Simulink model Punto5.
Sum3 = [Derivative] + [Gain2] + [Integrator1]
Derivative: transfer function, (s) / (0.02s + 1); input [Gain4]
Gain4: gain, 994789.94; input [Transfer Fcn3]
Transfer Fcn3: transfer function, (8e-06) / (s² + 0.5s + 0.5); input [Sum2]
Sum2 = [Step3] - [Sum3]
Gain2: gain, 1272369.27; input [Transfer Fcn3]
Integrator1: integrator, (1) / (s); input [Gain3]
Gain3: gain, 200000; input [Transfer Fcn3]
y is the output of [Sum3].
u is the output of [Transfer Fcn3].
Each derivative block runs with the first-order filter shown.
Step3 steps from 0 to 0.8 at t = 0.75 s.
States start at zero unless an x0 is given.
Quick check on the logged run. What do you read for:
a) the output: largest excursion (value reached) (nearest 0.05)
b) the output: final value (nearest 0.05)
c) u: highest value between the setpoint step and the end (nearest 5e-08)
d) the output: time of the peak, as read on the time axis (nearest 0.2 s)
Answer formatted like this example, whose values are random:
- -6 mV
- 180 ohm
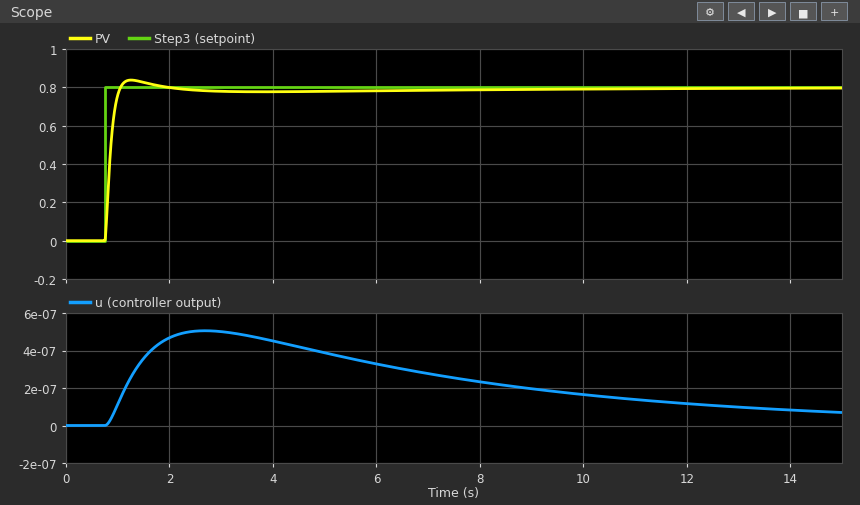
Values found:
- 0.85
- 0.80
- 0.00000050
- 1.2 s
